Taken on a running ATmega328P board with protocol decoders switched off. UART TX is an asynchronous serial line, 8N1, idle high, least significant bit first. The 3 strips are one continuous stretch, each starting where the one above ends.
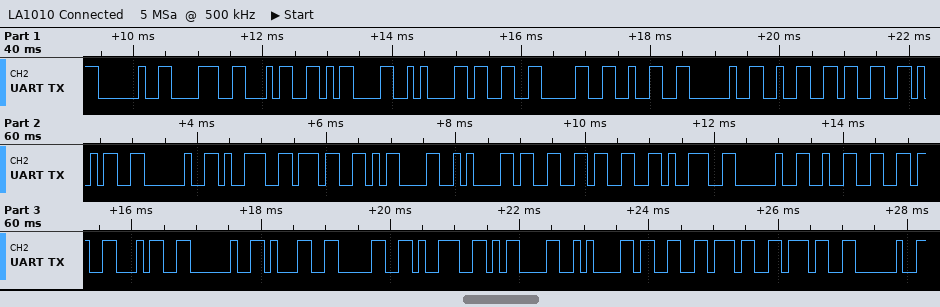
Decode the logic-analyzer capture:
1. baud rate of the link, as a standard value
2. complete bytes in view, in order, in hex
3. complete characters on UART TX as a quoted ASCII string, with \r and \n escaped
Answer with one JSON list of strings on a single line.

["9600 baud", "0x20 0x38 0x34 0x0D 0x0A 0x33 0x30 0x32 0x20 0x32 0x33 0x35 0x20 0x39 0x37 0x0D 0x0A 0x33 0x33 0x39 0x20 0x32 0x36 0x34 0x20 0x31 0x30 0x39 0x0D 0x0A 0x33 0x37 0x37 0x20", "\" 84\\r\\n302 235 97\\r\\n339 264 109\\r\\n377 \""]
